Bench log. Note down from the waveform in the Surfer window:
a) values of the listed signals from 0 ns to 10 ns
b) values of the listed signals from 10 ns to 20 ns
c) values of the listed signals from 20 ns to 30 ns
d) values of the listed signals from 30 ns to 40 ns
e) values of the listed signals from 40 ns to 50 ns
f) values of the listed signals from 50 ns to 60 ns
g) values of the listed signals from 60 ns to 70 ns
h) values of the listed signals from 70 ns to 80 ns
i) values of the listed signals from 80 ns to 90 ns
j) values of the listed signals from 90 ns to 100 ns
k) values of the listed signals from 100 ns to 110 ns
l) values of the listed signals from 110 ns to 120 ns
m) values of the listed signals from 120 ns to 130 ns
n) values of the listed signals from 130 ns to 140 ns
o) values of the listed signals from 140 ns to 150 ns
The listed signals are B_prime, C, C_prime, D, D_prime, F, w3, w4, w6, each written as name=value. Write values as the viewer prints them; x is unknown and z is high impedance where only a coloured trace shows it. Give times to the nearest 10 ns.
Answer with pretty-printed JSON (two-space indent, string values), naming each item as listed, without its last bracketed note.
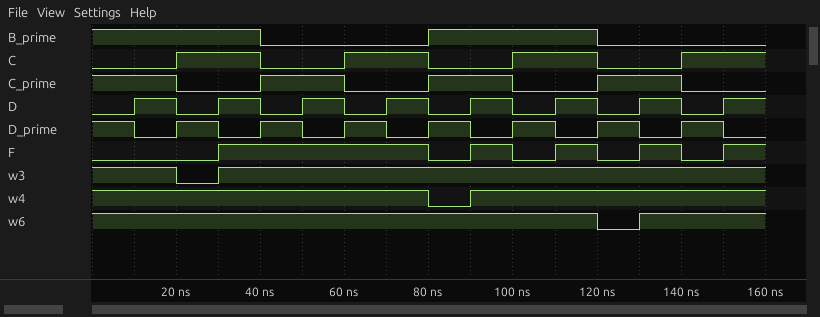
{
  "values of the listed signals from 0 ns to 10 ns": "B_prime=1, C=0, C_prime=1, D=0, D_prime=1, F=0, w3=1, w4=1, w6=1",
  "values of the listed signals from 10 ns to 20 ns": "B_prime=1, C=0, C_prime=1, D=1, D_prime=0, F=0, w3=1, w4=1, w6=1",
  "values of the listed signals from 20 ns to 30 ns": "B_prime=1, C=1, C_prime=0, D=0, D_prime=1, F=0, w3=0, w4=1, w6=1",
  "values of the listed signals from 30 ns to 40 ns": "B_prime=1, C=1, C_prime=0, D=1, D_prime=0, F=1, w3=1, w4=1, w6=1",
  "values of the listed signals from 40 ns to 50 ns": "B_prime=0, C=0, C_prime=1, D=0, D_prime=1, F=1, w3=1, w4=1, w6=1",
  "values of the listed signals from 50 ns to 60 ns": "B_prime=0, C=0, C_prime=1, D=1, D_prime=0, F=1, w3=1, w4=1, w6=1",
  "values of the listed signals from 60 ns to 70 ns": "B_prime=0, C=1, C_prime=0, D=0, D_prime=1, F=1, w3=1, w4=1, w6=1",
  "values of the listed signals from 70 ns to 80 ns": "B_prime=0, C=1, C_prime=0, D=1, D_prime=0, F=1, w3=1, w4=1, w6=1",
  "values of the listed signals from 80 ns to 90 ns": "B_prime=1, C=0, C_prime=1, D=0, D_prime=1, F=0, w3=1, w4=0, w6=1",
  "values of the listed signals from 90 ns to 100 ns": "B_prime=1, C=0, C_prime=1, D=1, D_prime=0, F=1, w3=1, w4=1, w6=1",
  "values of the listed signals from 100 ns to 110 ns": "B_prime=1, C=1, C_prime=0, D=0, D_prime=1, F=0, w3=1, w4=1, w6=1",
  "values of the listed signals from 110 ns to 120 ns": "B_prime=1, C=1, C_prime=0, D=1, D_prime=0, F=1, w3=1, w4=1, w6=1",
  "values of the listed signals from 120 ns to 130 ns": "B_prime=0, C=0, C_prime=1, D=0, D_prime=1, F=0, w3=1, w4=1, w6=0",
  "values of the listed signals from 130 ns to 140 ns": "B_prime=0, C=0, C_prime=1, D=1, D_prime=0, F=1, w3=1, w4=1, w6=1",
  "values of the listed signals from 140 ns to 150 ns": "B_prime=0, C=1, C_prime=0, D=0, D_prime=1, F=0, w3=1, w4=1, w6=1"
}
